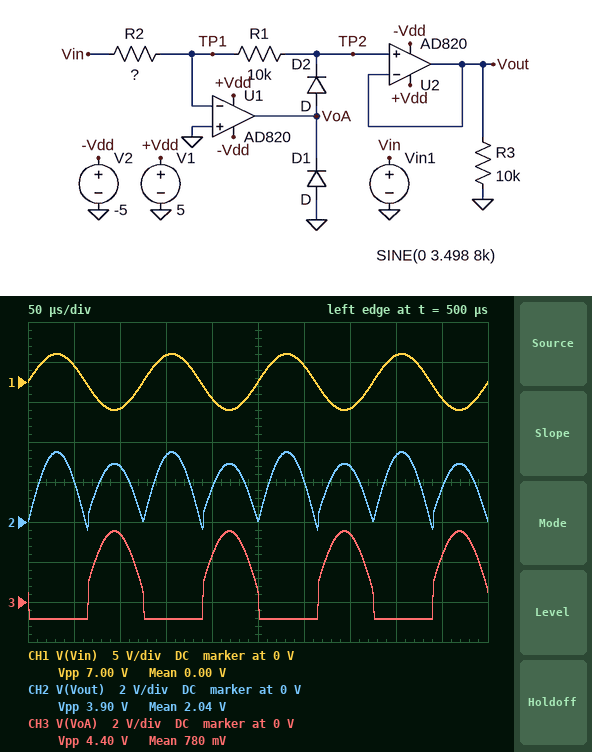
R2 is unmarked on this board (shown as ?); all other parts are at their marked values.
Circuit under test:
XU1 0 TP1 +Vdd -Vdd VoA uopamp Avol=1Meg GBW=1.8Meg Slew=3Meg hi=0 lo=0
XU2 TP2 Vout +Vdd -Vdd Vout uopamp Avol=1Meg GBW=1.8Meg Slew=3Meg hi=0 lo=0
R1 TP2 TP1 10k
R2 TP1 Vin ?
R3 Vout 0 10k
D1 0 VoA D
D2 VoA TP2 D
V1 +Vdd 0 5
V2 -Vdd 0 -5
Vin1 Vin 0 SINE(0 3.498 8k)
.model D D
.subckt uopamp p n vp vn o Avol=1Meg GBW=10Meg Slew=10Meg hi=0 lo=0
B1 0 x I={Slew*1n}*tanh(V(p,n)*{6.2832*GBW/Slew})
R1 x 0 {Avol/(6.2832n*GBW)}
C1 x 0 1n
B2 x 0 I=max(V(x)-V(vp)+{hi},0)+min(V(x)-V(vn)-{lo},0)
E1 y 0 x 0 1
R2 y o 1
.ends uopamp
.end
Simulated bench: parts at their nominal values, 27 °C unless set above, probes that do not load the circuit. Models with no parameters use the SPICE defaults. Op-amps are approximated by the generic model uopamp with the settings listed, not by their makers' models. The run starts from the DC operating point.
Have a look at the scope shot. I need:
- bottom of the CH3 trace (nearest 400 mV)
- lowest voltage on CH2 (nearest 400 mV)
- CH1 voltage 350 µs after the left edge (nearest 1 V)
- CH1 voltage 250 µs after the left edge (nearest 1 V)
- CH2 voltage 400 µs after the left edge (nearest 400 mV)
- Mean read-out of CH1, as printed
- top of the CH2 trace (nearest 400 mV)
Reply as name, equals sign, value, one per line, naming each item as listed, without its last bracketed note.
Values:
bottom of the CH3 trace = -800 mV
lowest voltage on CH2 = -400 mV
CH1 voltage 350 µs after the left edge = -3 V
CH1 voltage 250 µs after the left edge = 0 V
CH2 voltage 400 µs after the left edge = 3.2 V
Mean read-out of CH1, as printed = 0.00 V
top of the CH2 trace = 3.6 V
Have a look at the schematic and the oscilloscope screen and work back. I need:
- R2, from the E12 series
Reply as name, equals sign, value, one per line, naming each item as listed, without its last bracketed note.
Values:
R2, from the E12 series = 12 kΩ
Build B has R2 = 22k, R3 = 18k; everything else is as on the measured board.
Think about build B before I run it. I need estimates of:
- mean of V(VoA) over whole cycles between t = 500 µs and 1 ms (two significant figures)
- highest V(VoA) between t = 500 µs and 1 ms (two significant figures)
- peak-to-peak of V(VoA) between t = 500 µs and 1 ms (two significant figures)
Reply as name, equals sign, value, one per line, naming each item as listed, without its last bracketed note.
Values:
mean of V(VoA) over whole cycles between t = 500 µs and 1 ms = 340 mV
highest V(VoA) between t = 500 µs and 1 ms = 2.2 V
peak-to-peak of V(VoA) between t = 500 µs and 1 ms = 3.1 V
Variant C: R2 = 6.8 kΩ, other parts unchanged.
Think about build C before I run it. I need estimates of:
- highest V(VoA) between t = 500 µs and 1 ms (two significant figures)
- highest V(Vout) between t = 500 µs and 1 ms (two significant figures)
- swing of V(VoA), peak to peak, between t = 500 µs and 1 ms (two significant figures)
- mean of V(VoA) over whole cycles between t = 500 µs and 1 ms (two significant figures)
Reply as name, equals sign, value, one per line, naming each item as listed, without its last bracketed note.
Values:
highest V(VoA) between t = 500 µs and 1 ms = 5.0 V
highest V(Vout) between t = 500 µs and 1 ms = 4.4 V
swing of V(VoA), peak to peak, between t = 500 µs and 1 ms = 5.9 V
mean of V(VoA) over whole cycles between t = 500 µs and 1 ms = 1.4 V
